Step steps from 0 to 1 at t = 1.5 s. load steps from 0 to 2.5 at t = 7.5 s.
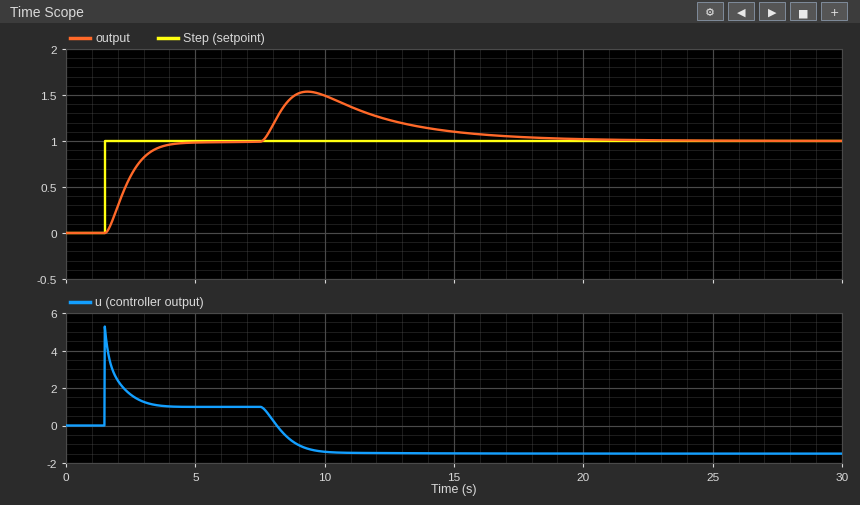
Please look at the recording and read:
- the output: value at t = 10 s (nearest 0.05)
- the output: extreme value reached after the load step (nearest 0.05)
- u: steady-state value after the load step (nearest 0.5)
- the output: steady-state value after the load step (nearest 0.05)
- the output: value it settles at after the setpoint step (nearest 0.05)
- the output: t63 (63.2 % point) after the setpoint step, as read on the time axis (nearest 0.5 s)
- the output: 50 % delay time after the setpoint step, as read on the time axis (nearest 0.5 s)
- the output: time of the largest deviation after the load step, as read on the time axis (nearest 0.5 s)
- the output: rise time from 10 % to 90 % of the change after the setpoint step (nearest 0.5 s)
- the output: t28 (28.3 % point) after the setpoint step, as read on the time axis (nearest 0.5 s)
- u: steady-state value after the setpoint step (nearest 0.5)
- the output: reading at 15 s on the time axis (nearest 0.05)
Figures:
1.50
1.55
-1.5
1.00
1.00
2.5 s
2.5 s
9.5 s
1.5 s
2.0 s
1.0
1.10
